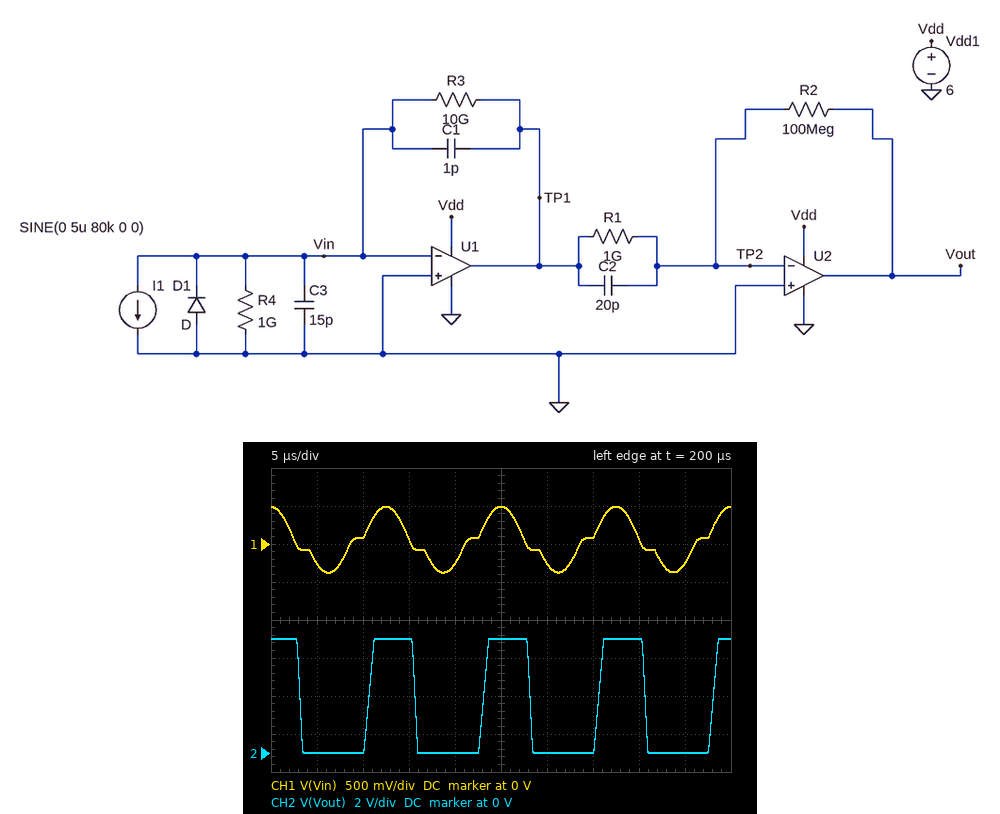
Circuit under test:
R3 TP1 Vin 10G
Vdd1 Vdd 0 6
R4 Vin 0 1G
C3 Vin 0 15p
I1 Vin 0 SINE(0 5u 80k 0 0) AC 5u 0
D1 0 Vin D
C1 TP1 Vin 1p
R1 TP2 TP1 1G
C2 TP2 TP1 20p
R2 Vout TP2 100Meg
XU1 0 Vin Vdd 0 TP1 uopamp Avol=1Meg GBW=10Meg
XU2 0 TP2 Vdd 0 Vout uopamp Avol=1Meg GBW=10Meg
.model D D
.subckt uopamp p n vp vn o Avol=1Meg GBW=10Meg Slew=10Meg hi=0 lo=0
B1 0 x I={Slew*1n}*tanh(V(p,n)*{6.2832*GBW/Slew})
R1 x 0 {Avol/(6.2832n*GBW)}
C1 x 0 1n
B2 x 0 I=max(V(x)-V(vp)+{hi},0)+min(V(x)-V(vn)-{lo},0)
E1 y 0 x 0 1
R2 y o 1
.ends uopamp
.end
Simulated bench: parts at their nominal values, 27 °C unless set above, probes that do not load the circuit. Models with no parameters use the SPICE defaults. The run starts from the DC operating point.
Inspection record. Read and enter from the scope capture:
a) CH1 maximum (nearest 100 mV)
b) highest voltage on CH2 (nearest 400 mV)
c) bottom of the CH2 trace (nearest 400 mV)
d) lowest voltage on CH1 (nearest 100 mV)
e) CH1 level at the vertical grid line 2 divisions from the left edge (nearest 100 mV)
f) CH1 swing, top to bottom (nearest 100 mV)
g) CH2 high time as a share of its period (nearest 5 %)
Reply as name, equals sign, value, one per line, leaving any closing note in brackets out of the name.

CH1 maximum = 500 mV
highest voltage on CH2 = 6.0 V
bottom of the CH2 trace = 0 V
lowest voltage on CH1 = -400 mV
CH1 level at the vertical grid line 2 divisions from the left edge = 100 mV
CH1 swing, top to bottom = 900 mV
CH2 high time as a share of its period = 40 %
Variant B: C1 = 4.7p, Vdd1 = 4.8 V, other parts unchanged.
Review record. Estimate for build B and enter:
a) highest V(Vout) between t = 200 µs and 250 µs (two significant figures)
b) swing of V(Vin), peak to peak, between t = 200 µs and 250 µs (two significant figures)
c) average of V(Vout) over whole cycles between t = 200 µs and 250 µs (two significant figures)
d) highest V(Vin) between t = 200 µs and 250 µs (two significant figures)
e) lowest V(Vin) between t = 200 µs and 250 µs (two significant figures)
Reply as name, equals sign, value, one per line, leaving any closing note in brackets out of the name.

highest V(Vout) between t = 200 µs and 250 µs = 4.8 V
swing of V(Vin), peak to peak, between t = 200 µs and 250 µs = 34 mV
average of V(Vout) over whole cycles between t = 200 µs and 250 µs = 620 mV
highest V(Vin) between t = 200 µs and 250 µs = 17 mV
lowest V(Vin) between t = 200 µs and 250 µs = -17 mV
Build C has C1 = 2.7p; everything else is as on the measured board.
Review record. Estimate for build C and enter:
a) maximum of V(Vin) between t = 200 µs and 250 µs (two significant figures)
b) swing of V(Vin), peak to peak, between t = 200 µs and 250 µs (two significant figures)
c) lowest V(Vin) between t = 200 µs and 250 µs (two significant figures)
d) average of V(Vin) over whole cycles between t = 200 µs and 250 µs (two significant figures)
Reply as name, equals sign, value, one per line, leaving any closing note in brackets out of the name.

maximum of V(Vin) between t = 200 µs and 250 µs = 30 mV
swing of V(Vin), peak to peak, between t = 200 µs and 250 µs = 230 mV
lowest V(Vin) between t = 200 µs and 250 µs = -200 mV
average of V(Vin) over whole cycles between t = 200 µs and 250 µs = -37 mV
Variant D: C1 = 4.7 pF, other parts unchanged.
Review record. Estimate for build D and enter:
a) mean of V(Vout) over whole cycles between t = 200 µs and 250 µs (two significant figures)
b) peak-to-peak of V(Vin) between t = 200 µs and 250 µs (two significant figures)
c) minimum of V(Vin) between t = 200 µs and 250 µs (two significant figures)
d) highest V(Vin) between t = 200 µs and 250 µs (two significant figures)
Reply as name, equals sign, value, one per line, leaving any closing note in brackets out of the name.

mean of V(Vout) over whole cycles between t = 200 µs and 250 µs = 760 mV
peak-to-peak of V(Vin) between t = 200 µs and 250 µs = 34 mV
minimum of V(Vin) between t = 200 µs and 250 µs = -17 mV
highest V(Vin) between t = 200 µs and 250 µs = 17 mV
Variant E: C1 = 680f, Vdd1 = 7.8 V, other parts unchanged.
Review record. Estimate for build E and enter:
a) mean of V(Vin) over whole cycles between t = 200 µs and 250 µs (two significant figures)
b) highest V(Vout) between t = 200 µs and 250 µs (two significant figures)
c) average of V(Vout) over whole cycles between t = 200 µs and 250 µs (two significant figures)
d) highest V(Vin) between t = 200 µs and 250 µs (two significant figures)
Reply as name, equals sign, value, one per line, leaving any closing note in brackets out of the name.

mean of V(Vin) over whole cycles between t = 200 µs and 250 µs = 73 mV
highest V(Vout) between t = 200 µs and 250 µs = 7.8 V
average of V(Vout) over whole cycles between t = 200 µs and 250 µs = 3.2 V
highest V(Vin) between t = 200 µs and 250 µs = 560 mV
